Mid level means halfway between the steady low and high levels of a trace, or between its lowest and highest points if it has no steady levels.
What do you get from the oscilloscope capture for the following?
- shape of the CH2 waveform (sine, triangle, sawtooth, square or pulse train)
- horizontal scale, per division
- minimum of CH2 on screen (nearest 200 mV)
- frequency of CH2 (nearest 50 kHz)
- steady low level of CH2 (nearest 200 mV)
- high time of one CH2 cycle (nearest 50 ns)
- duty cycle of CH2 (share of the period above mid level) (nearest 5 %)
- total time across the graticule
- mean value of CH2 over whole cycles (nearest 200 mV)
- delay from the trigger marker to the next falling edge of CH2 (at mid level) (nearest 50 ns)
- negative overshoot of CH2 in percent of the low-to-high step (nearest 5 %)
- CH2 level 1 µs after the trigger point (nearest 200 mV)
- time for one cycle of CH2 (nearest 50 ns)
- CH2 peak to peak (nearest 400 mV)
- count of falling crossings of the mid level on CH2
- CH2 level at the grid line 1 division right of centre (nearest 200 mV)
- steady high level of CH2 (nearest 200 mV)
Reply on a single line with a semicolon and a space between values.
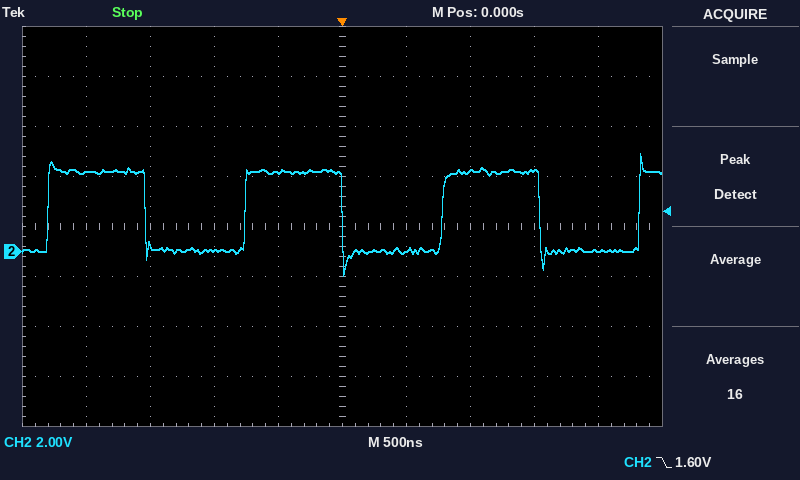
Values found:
square; 500 ns; -1.0 V; 650 kHz; 0.0 V; 750 ns; 50 %; 5 µs; 1.6 V; 1.55 µs; 30 %; 3.2 V; 1.55 µs; 4.8 V; 3; 0.0 V; 3.2 V
